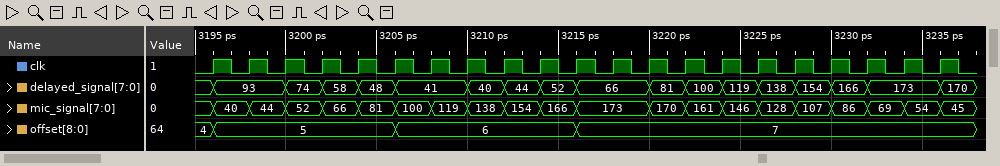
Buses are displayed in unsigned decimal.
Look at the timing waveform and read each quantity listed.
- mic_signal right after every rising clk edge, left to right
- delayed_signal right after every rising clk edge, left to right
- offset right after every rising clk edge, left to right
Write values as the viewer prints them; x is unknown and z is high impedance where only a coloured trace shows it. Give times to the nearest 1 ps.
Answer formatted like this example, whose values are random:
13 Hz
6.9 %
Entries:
40, 44, 52, 66, 81, 100, 119, 138, 154, 166, 173, 173, 170, 161, 146, 128, 107, 86, 69, 54, 45
93, 93, 74, 58, 48, 41, 41, 40, 44, 52, 66, 66, 81, 100, 119, 138, 154, 166, 173, 173, 170
5, 5, 5, 5, 5, 6, 6, 6, 6, 6, 7, 7, 7, 7, 7, 7, 7, 7, 7, 7, 7
